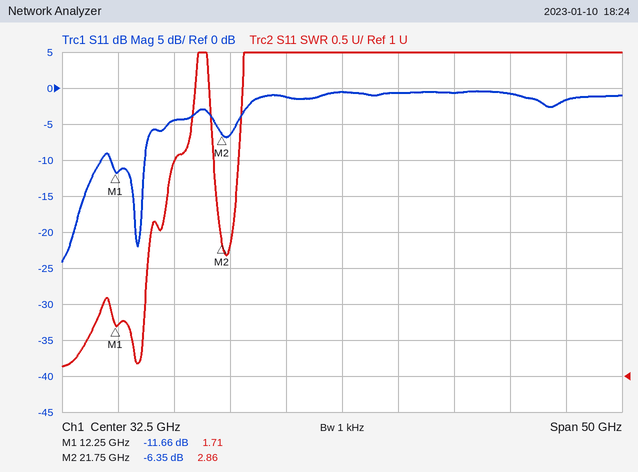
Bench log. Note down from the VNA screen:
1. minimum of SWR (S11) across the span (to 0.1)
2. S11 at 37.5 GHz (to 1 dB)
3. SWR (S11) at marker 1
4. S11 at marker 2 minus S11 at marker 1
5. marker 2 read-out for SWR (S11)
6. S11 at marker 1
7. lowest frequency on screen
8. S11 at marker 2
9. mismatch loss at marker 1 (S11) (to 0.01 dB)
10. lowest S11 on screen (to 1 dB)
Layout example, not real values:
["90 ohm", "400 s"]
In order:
["1.1", "-1 dB", "1.71", "5.31 dB", "2.86", "-11.66 dB", "7.5 GHz", "-6.35 dB", "0.31 dB", "-24 dB"]
